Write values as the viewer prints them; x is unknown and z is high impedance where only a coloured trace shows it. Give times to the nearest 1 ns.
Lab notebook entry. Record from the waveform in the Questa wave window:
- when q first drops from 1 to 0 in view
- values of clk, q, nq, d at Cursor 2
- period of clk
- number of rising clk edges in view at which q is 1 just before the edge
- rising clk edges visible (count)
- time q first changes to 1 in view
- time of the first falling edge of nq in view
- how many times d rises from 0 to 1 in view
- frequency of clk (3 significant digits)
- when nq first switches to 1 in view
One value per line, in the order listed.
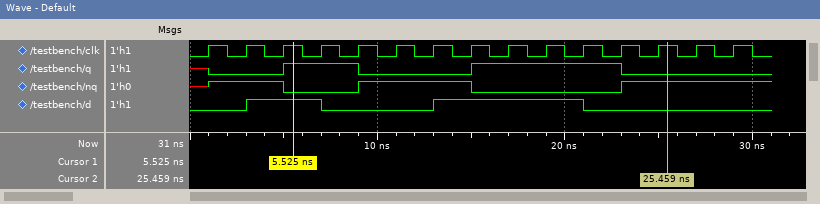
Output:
9 ns
clk=1, q=0, nq=1, d=0
2 ns
6
15
5 ns
5 ns
2
500 MHz
1 ns
